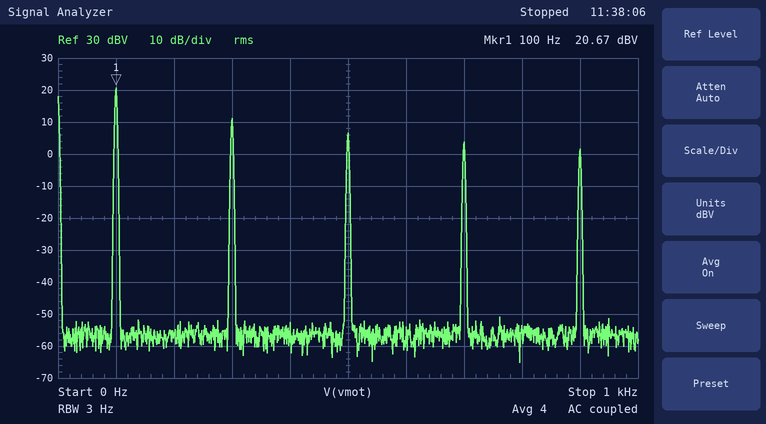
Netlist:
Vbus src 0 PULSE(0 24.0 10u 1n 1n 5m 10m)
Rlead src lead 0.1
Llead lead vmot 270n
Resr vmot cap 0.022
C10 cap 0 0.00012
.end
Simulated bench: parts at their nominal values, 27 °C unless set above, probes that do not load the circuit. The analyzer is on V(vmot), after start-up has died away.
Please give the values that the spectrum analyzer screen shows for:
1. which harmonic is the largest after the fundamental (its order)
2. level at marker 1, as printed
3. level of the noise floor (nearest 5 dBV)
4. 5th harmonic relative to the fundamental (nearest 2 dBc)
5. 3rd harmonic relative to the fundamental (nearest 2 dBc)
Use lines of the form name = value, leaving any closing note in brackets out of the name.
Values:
which harmonic is the largest after the fundamental = 3
level at marker 1, as printed = 20.67 dBV
level of the noise floor = -55 dBV
5th harmonic relative to the fundamental = -14 dBc
3rd harmonic relative to the fundamental = -10 dBc
